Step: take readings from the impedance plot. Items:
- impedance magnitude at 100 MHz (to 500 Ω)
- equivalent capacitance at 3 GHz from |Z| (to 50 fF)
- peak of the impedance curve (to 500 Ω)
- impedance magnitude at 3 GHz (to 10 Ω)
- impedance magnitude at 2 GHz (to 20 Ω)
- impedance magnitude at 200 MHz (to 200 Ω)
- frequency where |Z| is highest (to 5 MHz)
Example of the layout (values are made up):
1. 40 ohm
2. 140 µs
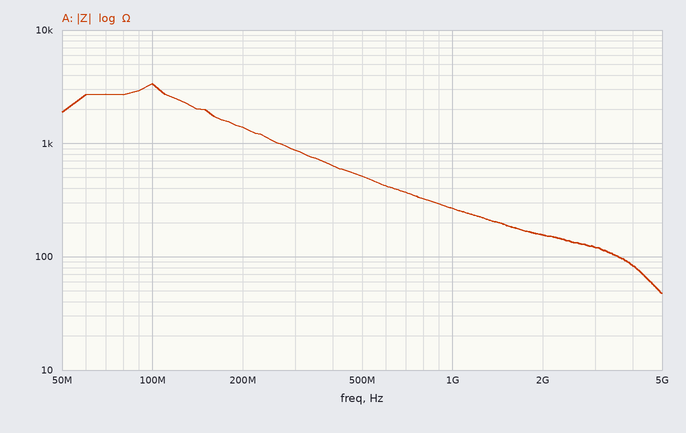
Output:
1. 3.5 kΩ
2. 450 fF
3. 3.5 kΩ
4. 120 Ω
5. 160 Ω
6. 1.4 kΩ
7. 100 MHz
